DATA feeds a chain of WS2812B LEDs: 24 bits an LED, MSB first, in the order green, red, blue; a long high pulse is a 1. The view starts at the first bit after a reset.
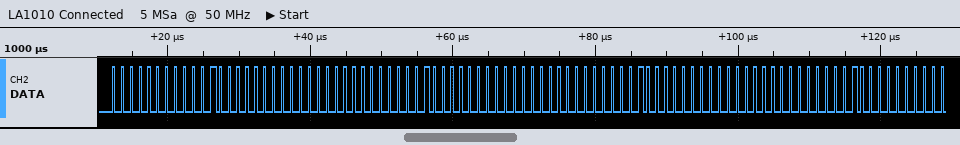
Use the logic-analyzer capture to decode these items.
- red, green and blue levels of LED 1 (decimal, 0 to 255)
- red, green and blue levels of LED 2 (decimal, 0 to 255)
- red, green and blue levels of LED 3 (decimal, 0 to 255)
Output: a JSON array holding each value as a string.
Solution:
["16, 0, 0", "16, 0, 0", "16, 0, 0"]
